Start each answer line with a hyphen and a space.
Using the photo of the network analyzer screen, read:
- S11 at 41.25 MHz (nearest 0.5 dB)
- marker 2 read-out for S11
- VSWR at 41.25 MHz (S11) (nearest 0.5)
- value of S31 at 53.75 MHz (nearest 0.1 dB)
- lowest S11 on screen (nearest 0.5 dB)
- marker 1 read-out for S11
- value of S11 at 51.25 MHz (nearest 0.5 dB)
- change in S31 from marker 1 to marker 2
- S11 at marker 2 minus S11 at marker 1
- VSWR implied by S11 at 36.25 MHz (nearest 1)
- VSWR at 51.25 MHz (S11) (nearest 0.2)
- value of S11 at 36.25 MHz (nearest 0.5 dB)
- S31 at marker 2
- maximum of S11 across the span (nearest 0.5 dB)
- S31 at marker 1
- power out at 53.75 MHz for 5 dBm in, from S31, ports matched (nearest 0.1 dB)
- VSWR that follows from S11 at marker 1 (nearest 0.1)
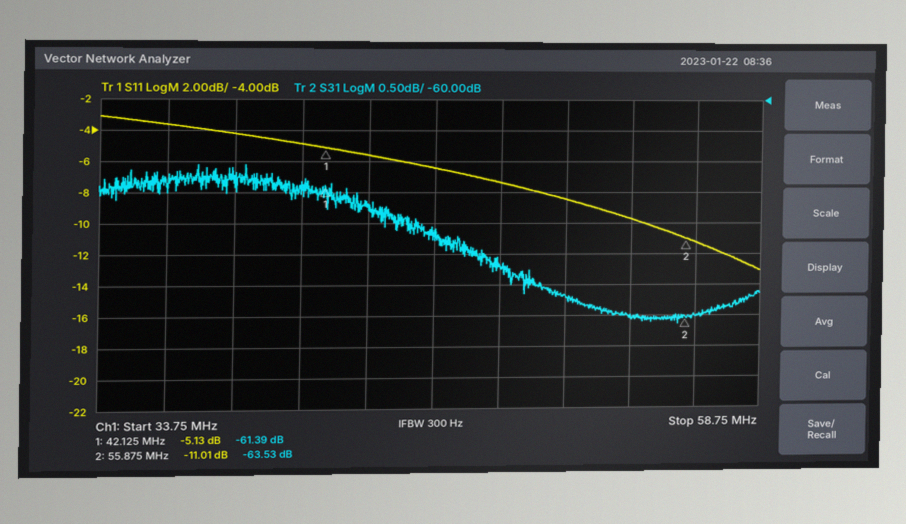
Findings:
- -5.0 dB
- -11.01 dB
- 3.5
- -63.5 dB
- -13.0 dB
- -5.13 dB
- -8.5 dB
- -2.14 dB
- -5.88 dB
- 5
- 2.2
- -3.5 dB
- -63.53 dB
- -3.0 dB
- -61.39 dB
- -58.5 dBm
- 3.5
